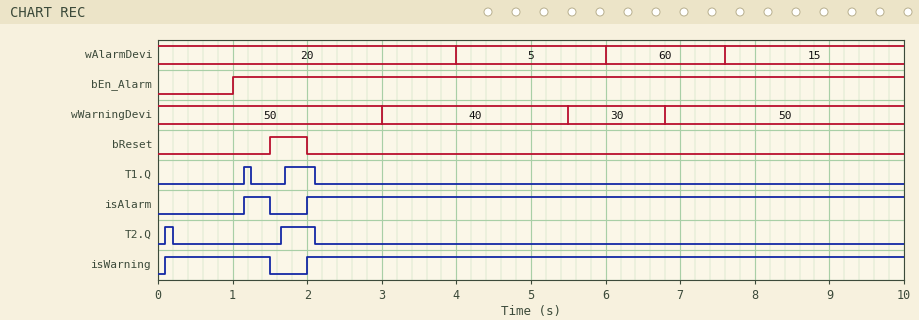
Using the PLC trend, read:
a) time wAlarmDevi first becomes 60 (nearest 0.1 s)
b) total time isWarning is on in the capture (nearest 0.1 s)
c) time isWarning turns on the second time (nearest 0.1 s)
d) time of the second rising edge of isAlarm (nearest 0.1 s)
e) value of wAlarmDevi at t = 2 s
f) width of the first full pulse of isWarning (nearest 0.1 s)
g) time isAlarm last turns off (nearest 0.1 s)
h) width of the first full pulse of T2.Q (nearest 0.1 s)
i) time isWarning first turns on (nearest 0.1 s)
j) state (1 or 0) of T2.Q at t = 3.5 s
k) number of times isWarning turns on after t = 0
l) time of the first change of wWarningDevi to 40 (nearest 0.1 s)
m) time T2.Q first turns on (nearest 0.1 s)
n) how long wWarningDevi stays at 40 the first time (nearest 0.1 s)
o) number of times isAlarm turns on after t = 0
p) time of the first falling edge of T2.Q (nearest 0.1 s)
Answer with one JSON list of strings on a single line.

["6.0 s", "9.4 s", "2.0 s", "2.0 s", "20", "1.4 s", "1.5 s", "0.1 s", "0.1 s", "0", "2", "3.0 s", "0.1 s", "2.5 s", "2", "0.2 s"]
